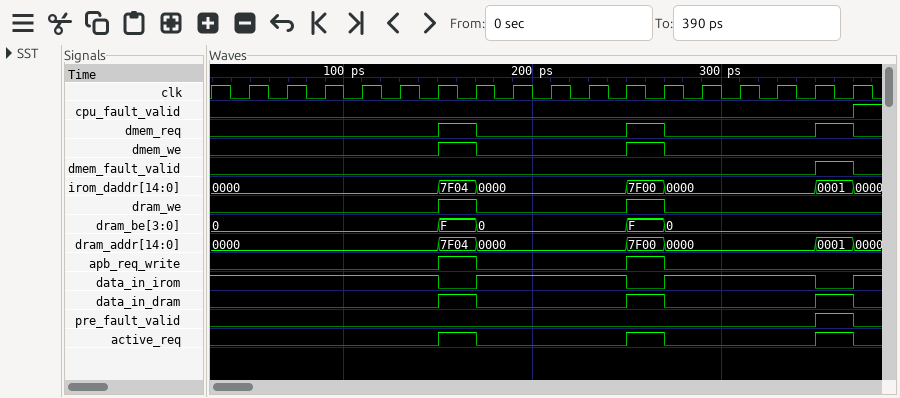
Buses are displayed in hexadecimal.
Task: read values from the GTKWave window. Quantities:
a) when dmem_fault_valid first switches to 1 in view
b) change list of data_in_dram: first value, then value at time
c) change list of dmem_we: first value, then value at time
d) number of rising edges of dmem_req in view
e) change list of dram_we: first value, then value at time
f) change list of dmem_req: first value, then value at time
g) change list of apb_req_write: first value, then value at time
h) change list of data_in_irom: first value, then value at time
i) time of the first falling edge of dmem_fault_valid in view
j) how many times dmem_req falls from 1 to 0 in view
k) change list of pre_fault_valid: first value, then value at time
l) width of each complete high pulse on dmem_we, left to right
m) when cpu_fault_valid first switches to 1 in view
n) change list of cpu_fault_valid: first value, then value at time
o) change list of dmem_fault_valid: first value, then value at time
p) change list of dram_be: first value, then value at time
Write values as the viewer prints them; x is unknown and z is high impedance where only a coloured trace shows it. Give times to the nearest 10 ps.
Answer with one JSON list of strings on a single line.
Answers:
["350 ps", "0, 1 at 150 ps, 0 at 170 ps, 1 at 250 ps, 0 at 270 ps, 1 at 350 ps, 0 at 370 ps", "0, 1 at 150 ps, 0 at 170 ps, 1 at 250 ps, 0 at 270 ps", "3", "0, 1 at 150 ps, 0 at 170 ps, 1 at 250 ps, 0 at 270 ps", "0, 1 at 150 ps, 0 at 170 ps, 1 at 250 ps, 0 at 270 ps, 1 at 350 ps, 0 at 370 ps", "0, 1 at 150 ps, 0 at 170 ps, 1 at 250 ps, 0 at 270 ps", "1, 0 at 150 ps, 1 at 170 ps, 0 at 250 ps, 1 at 270 ps, 0 at 350 ps, 1 at 370 ps", "370 ps", "3", "0, 1 at 350 ps, 0 at 370 ps", "20 ps, 20 ps", "370 ps", "0, 1 at 370 ps", "0, 1 at 350 ps, 0 at 370 ps", "0, F at 150 ps, 0 at 170 ps, F at 250 ps, 0 at 270 ps"]
